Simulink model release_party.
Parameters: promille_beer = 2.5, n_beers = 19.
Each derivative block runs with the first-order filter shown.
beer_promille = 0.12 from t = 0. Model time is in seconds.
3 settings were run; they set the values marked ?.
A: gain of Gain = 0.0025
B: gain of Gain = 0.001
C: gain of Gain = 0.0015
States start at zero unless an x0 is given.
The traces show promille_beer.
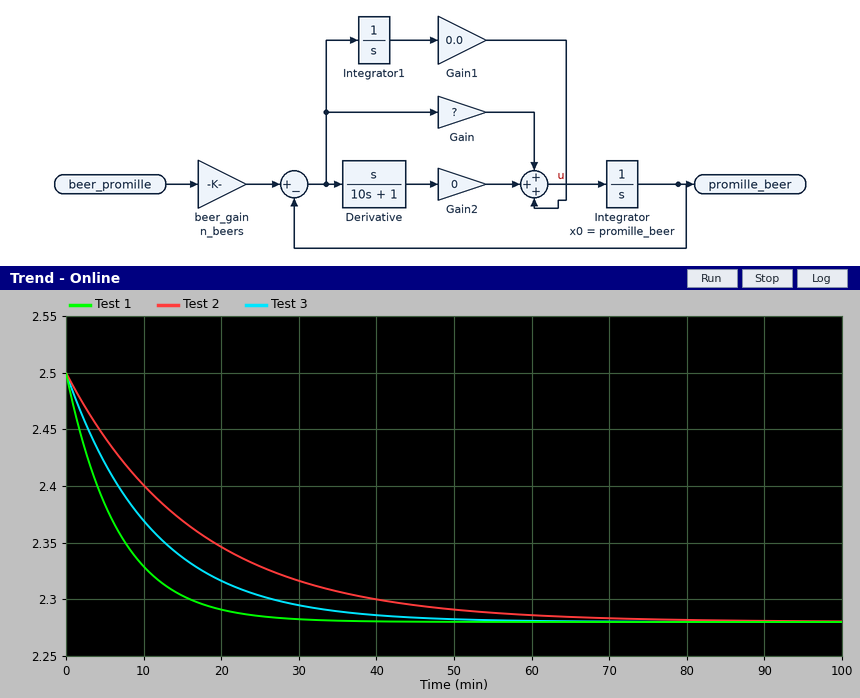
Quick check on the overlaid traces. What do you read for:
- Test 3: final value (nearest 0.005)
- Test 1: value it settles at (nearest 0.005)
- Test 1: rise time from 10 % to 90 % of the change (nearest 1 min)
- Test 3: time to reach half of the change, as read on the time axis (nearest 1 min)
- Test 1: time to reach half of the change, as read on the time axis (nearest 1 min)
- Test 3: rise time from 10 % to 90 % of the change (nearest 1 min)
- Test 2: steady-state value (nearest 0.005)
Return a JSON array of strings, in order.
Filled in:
["2.280", "2.280", "15 min", "8 min", "5 min", "24 min", "2.280"]
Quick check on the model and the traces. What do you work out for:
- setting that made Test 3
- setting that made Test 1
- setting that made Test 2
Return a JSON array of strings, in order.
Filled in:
["C", "A", "B"]
